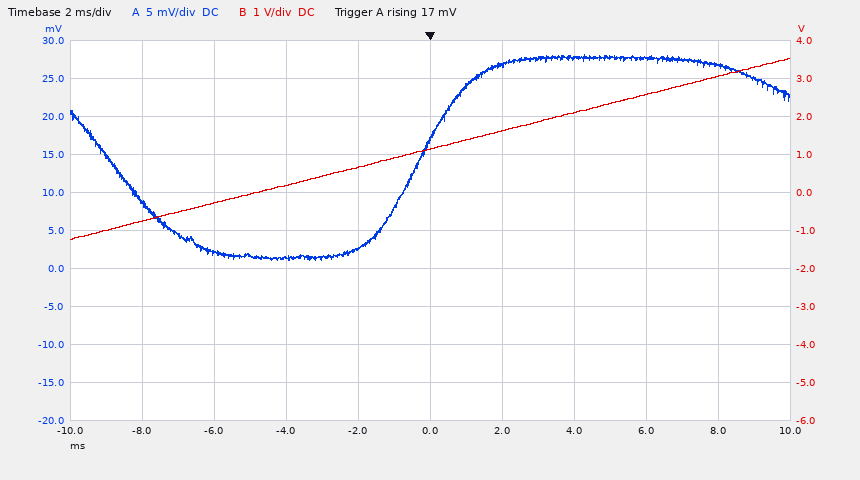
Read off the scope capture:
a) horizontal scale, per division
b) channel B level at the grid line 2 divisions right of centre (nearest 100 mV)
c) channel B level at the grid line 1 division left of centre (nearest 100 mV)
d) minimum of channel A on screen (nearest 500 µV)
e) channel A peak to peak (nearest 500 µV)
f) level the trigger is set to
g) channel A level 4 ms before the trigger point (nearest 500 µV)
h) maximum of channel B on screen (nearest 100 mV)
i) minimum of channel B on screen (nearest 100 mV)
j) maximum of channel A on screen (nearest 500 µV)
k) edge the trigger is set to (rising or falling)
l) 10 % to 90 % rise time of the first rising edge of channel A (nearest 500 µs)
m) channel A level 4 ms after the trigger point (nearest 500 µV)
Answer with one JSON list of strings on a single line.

["2 ms", "2.1 V", "700 mV", "1.0 mV", "27.0 mV", "17 mV", "1.5 mV", "3.5 V", "-1.2 V", "28.0 mV", "rising", "3.0 ms", "27.5 mV"]
